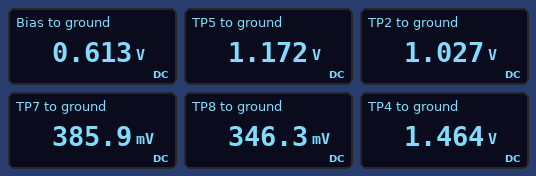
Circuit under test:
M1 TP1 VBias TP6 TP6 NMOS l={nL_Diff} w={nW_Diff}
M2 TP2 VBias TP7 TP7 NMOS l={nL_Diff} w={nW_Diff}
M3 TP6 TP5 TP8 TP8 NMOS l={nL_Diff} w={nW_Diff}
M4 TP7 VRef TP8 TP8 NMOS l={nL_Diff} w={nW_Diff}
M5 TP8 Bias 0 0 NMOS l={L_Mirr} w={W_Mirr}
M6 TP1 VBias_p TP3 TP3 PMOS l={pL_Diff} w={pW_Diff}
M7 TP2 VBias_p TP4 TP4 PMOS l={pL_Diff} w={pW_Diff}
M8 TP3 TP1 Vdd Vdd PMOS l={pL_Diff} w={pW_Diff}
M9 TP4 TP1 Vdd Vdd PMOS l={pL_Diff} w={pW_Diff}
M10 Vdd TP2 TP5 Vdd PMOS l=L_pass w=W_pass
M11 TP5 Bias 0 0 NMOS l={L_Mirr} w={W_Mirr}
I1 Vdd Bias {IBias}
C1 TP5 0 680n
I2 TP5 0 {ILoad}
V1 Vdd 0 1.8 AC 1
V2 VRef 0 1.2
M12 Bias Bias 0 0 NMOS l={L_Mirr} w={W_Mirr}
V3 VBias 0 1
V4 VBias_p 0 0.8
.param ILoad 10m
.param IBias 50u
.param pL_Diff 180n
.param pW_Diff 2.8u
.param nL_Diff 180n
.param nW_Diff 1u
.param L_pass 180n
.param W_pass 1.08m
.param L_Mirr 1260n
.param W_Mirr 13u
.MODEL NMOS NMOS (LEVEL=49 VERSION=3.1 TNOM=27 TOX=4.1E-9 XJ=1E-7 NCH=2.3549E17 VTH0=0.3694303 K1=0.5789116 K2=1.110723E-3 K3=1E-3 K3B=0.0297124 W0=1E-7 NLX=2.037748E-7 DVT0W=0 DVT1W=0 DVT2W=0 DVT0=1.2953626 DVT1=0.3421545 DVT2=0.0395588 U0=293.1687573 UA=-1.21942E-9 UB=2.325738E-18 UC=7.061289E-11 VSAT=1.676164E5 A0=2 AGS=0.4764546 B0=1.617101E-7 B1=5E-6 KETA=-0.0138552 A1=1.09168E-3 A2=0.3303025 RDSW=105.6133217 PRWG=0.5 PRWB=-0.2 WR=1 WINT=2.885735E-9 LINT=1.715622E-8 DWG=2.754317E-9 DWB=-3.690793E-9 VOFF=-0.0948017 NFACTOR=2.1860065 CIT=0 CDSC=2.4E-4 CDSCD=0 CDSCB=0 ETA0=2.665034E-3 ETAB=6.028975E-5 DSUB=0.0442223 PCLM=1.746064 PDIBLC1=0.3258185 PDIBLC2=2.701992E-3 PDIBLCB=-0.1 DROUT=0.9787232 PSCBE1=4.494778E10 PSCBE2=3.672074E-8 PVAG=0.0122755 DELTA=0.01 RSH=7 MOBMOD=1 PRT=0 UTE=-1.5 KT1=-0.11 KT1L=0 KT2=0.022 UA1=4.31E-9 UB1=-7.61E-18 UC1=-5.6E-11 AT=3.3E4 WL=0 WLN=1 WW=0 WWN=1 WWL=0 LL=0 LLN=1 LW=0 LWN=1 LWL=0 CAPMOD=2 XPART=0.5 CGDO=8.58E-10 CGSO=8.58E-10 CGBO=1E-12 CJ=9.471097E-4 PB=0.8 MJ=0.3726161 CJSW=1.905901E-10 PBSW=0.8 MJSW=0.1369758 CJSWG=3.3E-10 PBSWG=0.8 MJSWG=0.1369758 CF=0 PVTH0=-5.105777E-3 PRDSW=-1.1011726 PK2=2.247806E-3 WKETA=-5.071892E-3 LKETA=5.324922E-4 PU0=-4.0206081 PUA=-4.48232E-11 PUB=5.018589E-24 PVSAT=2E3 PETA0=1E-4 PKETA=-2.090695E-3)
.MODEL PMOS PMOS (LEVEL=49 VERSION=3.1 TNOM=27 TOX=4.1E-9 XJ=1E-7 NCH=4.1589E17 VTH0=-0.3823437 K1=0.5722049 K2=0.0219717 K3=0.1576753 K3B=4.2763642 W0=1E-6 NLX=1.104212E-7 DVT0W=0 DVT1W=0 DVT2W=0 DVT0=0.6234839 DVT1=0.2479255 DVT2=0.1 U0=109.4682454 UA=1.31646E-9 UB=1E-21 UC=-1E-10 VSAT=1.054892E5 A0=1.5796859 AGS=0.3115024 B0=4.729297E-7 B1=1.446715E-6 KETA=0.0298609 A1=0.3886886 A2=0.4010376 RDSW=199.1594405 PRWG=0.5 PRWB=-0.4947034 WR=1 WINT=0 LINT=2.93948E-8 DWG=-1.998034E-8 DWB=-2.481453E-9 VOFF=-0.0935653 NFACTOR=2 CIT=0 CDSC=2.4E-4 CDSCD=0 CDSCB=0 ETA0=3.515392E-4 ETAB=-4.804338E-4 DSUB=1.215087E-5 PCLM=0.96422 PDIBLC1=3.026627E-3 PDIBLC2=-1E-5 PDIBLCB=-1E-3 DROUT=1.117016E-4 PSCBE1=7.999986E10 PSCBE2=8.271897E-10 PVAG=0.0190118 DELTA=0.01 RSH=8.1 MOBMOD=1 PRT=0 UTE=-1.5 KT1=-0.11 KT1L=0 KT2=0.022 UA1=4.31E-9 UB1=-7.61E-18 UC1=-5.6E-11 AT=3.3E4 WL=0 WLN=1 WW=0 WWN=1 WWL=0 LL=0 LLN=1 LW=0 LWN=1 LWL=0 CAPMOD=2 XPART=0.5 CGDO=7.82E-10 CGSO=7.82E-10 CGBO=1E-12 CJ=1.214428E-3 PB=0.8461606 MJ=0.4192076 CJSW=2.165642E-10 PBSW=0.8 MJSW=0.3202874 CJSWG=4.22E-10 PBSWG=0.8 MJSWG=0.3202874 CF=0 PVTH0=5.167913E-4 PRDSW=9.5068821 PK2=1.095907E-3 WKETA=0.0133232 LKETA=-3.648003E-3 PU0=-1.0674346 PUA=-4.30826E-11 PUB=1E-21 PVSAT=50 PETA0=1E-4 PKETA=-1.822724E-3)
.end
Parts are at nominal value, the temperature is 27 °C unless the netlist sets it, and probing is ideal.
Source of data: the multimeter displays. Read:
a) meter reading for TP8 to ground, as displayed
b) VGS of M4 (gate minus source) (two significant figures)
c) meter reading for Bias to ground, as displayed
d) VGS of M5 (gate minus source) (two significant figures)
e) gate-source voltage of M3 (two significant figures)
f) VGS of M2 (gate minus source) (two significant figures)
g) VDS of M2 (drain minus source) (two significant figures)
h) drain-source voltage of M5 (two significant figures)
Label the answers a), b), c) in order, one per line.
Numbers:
a) 346.3 mV
b) 850 mV
c) 0.613 V
d) 610 mV
e) 830 mV
f) 610 mV
g) 640 mV
h) 350 mV
